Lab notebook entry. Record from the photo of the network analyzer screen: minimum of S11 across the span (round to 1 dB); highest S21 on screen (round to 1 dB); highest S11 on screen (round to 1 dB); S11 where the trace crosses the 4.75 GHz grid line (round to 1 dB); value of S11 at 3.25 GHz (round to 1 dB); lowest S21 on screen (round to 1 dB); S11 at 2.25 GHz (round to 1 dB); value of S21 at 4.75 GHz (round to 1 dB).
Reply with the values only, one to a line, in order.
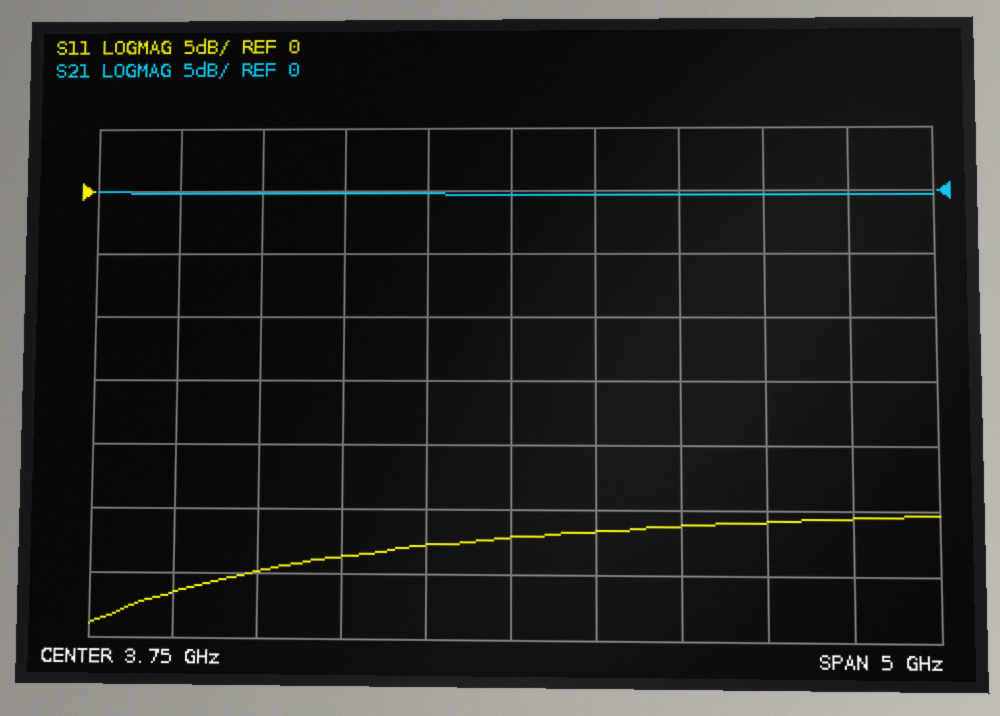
-34 dB
0 dB
-25 dB
-26 dB
-28 dB
0 dB
-30 dB
0 dB
